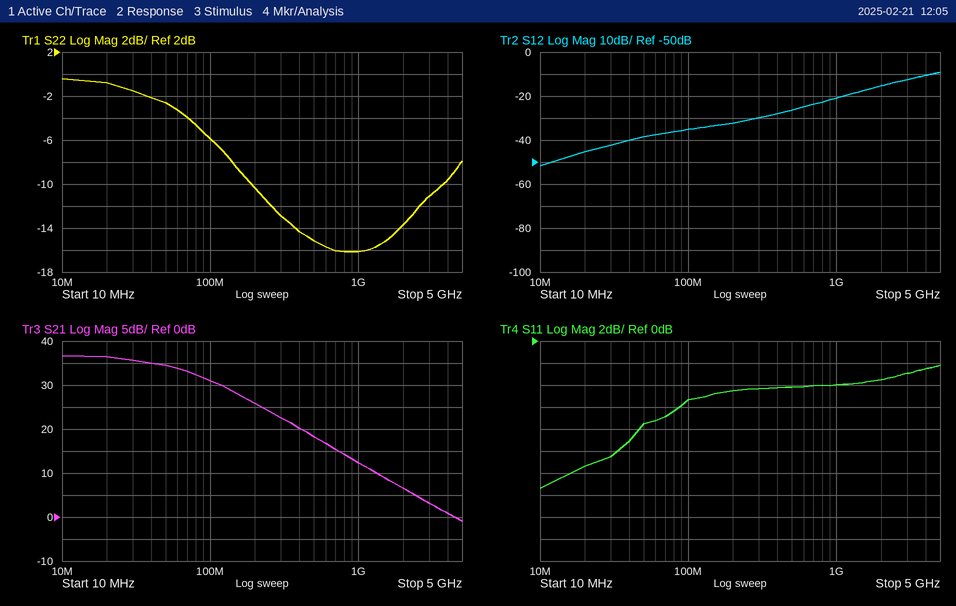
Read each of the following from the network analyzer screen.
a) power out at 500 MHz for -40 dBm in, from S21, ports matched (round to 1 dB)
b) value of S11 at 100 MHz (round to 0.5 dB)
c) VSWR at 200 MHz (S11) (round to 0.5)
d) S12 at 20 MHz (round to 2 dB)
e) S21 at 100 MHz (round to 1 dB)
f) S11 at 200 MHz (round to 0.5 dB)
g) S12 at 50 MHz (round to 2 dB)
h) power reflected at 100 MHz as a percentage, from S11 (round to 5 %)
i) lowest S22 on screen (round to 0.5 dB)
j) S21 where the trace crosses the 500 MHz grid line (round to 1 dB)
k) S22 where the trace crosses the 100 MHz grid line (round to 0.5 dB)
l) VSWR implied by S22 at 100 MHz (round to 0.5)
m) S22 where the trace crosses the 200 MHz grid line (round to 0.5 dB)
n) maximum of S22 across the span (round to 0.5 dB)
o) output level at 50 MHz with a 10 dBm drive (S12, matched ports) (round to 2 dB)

-22 dBm
-5.5 dB
4.0
-46 dB
31 dB
-4.5 dB
-38 dB
30 %
-16.0 dB
18 dB
-6.0 dB
3.0
-10.5 dB
-0.5 dB
-28 dBm
